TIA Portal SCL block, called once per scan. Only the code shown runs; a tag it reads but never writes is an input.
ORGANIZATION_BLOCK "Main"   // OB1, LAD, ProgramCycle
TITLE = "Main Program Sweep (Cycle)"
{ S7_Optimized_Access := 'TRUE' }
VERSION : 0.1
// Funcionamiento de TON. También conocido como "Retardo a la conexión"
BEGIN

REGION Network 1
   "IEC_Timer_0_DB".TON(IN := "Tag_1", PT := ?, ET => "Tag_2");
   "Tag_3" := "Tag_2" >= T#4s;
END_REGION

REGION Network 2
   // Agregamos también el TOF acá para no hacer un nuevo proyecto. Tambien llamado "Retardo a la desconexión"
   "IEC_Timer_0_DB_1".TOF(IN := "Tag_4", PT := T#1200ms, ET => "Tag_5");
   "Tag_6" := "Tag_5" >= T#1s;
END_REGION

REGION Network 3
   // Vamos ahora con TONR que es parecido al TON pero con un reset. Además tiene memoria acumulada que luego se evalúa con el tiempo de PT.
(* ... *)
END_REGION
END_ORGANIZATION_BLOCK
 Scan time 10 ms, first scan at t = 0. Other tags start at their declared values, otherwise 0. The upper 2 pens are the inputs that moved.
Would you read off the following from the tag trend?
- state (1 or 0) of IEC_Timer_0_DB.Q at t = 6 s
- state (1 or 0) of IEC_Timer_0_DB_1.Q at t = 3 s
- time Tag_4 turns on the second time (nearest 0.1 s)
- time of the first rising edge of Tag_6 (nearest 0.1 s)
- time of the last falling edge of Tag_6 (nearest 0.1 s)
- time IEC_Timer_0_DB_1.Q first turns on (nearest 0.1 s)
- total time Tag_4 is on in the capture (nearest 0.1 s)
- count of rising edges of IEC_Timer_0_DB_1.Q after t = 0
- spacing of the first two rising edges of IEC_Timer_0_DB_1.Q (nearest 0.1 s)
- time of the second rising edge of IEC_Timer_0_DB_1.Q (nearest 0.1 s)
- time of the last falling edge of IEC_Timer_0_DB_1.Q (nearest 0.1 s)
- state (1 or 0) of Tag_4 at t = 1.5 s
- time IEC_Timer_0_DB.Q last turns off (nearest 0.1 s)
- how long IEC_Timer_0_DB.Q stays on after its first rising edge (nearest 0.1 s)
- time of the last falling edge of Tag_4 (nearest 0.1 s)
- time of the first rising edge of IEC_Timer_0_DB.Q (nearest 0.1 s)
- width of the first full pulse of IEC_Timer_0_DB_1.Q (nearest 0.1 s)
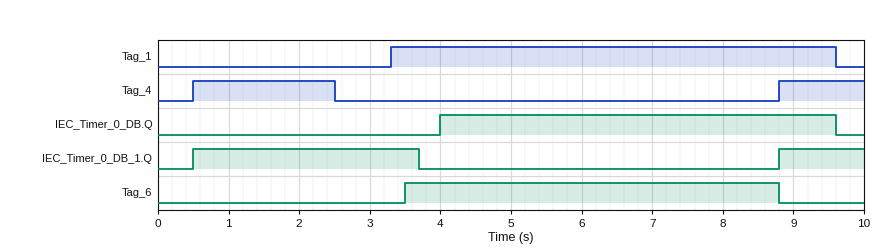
1
1
8.8 s
3.5 s
8.8 s
0.5 s
3.2 s
2
8.3 s
8.8 s
3.7 s
1
9.6 s
5.6 s
2.5 s
4.0 s
3.2 s
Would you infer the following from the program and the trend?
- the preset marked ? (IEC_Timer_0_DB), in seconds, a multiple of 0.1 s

0.7 s
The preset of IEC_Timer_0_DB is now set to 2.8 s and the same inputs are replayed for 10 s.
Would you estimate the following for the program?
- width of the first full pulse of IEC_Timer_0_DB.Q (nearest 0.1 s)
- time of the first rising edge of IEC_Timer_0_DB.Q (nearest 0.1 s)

3.5 s
6.1 s
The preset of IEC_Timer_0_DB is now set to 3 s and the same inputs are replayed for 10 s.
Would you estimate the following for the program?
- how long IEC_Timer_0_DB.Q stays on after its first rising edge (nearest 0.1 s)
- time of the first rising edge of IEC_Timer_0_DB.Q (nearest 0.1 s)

3.3 s
6.3 s
